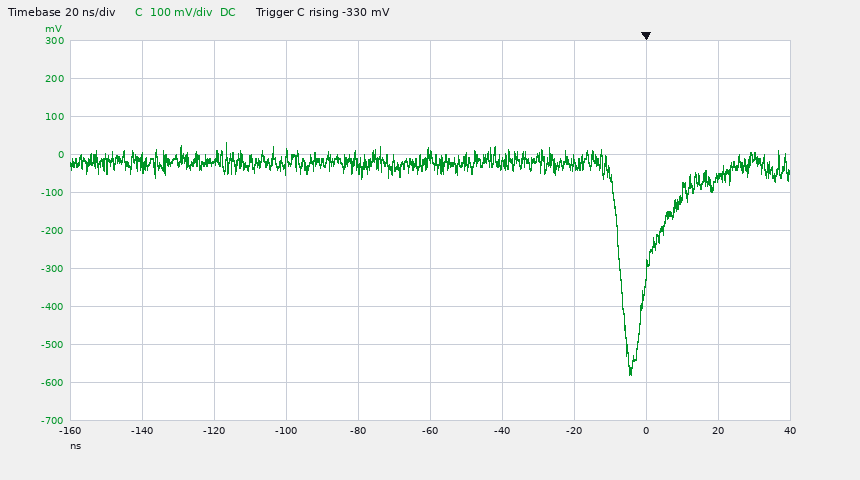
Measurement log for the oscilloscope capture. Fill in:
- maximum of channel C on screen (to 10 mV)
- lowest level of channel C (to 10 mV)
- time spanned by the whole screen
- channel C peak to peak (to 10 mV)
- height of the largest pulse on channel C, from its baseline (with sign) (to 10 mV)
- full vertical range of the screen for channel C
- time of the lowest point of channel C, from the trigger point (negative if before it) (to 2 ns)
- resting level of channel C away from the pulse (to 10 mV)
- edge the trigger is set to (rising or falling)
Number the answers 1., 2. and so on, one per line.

1. 30 mV
2. -580 mV
3. 200 ns
4. 610 mV
5. -560 mV
6. 1 V
7. -4 ns
8. -20 mV
9. rising
